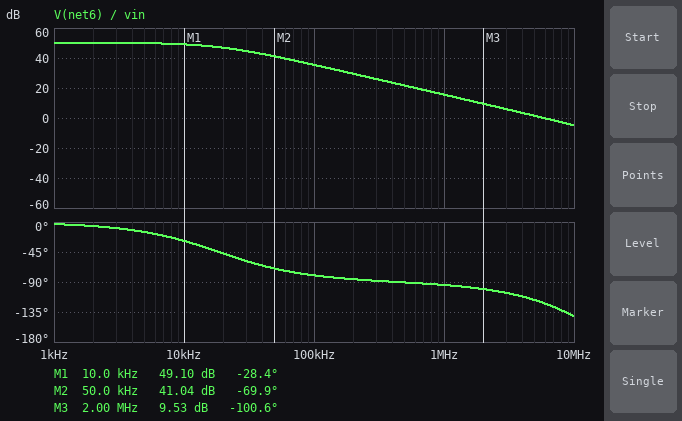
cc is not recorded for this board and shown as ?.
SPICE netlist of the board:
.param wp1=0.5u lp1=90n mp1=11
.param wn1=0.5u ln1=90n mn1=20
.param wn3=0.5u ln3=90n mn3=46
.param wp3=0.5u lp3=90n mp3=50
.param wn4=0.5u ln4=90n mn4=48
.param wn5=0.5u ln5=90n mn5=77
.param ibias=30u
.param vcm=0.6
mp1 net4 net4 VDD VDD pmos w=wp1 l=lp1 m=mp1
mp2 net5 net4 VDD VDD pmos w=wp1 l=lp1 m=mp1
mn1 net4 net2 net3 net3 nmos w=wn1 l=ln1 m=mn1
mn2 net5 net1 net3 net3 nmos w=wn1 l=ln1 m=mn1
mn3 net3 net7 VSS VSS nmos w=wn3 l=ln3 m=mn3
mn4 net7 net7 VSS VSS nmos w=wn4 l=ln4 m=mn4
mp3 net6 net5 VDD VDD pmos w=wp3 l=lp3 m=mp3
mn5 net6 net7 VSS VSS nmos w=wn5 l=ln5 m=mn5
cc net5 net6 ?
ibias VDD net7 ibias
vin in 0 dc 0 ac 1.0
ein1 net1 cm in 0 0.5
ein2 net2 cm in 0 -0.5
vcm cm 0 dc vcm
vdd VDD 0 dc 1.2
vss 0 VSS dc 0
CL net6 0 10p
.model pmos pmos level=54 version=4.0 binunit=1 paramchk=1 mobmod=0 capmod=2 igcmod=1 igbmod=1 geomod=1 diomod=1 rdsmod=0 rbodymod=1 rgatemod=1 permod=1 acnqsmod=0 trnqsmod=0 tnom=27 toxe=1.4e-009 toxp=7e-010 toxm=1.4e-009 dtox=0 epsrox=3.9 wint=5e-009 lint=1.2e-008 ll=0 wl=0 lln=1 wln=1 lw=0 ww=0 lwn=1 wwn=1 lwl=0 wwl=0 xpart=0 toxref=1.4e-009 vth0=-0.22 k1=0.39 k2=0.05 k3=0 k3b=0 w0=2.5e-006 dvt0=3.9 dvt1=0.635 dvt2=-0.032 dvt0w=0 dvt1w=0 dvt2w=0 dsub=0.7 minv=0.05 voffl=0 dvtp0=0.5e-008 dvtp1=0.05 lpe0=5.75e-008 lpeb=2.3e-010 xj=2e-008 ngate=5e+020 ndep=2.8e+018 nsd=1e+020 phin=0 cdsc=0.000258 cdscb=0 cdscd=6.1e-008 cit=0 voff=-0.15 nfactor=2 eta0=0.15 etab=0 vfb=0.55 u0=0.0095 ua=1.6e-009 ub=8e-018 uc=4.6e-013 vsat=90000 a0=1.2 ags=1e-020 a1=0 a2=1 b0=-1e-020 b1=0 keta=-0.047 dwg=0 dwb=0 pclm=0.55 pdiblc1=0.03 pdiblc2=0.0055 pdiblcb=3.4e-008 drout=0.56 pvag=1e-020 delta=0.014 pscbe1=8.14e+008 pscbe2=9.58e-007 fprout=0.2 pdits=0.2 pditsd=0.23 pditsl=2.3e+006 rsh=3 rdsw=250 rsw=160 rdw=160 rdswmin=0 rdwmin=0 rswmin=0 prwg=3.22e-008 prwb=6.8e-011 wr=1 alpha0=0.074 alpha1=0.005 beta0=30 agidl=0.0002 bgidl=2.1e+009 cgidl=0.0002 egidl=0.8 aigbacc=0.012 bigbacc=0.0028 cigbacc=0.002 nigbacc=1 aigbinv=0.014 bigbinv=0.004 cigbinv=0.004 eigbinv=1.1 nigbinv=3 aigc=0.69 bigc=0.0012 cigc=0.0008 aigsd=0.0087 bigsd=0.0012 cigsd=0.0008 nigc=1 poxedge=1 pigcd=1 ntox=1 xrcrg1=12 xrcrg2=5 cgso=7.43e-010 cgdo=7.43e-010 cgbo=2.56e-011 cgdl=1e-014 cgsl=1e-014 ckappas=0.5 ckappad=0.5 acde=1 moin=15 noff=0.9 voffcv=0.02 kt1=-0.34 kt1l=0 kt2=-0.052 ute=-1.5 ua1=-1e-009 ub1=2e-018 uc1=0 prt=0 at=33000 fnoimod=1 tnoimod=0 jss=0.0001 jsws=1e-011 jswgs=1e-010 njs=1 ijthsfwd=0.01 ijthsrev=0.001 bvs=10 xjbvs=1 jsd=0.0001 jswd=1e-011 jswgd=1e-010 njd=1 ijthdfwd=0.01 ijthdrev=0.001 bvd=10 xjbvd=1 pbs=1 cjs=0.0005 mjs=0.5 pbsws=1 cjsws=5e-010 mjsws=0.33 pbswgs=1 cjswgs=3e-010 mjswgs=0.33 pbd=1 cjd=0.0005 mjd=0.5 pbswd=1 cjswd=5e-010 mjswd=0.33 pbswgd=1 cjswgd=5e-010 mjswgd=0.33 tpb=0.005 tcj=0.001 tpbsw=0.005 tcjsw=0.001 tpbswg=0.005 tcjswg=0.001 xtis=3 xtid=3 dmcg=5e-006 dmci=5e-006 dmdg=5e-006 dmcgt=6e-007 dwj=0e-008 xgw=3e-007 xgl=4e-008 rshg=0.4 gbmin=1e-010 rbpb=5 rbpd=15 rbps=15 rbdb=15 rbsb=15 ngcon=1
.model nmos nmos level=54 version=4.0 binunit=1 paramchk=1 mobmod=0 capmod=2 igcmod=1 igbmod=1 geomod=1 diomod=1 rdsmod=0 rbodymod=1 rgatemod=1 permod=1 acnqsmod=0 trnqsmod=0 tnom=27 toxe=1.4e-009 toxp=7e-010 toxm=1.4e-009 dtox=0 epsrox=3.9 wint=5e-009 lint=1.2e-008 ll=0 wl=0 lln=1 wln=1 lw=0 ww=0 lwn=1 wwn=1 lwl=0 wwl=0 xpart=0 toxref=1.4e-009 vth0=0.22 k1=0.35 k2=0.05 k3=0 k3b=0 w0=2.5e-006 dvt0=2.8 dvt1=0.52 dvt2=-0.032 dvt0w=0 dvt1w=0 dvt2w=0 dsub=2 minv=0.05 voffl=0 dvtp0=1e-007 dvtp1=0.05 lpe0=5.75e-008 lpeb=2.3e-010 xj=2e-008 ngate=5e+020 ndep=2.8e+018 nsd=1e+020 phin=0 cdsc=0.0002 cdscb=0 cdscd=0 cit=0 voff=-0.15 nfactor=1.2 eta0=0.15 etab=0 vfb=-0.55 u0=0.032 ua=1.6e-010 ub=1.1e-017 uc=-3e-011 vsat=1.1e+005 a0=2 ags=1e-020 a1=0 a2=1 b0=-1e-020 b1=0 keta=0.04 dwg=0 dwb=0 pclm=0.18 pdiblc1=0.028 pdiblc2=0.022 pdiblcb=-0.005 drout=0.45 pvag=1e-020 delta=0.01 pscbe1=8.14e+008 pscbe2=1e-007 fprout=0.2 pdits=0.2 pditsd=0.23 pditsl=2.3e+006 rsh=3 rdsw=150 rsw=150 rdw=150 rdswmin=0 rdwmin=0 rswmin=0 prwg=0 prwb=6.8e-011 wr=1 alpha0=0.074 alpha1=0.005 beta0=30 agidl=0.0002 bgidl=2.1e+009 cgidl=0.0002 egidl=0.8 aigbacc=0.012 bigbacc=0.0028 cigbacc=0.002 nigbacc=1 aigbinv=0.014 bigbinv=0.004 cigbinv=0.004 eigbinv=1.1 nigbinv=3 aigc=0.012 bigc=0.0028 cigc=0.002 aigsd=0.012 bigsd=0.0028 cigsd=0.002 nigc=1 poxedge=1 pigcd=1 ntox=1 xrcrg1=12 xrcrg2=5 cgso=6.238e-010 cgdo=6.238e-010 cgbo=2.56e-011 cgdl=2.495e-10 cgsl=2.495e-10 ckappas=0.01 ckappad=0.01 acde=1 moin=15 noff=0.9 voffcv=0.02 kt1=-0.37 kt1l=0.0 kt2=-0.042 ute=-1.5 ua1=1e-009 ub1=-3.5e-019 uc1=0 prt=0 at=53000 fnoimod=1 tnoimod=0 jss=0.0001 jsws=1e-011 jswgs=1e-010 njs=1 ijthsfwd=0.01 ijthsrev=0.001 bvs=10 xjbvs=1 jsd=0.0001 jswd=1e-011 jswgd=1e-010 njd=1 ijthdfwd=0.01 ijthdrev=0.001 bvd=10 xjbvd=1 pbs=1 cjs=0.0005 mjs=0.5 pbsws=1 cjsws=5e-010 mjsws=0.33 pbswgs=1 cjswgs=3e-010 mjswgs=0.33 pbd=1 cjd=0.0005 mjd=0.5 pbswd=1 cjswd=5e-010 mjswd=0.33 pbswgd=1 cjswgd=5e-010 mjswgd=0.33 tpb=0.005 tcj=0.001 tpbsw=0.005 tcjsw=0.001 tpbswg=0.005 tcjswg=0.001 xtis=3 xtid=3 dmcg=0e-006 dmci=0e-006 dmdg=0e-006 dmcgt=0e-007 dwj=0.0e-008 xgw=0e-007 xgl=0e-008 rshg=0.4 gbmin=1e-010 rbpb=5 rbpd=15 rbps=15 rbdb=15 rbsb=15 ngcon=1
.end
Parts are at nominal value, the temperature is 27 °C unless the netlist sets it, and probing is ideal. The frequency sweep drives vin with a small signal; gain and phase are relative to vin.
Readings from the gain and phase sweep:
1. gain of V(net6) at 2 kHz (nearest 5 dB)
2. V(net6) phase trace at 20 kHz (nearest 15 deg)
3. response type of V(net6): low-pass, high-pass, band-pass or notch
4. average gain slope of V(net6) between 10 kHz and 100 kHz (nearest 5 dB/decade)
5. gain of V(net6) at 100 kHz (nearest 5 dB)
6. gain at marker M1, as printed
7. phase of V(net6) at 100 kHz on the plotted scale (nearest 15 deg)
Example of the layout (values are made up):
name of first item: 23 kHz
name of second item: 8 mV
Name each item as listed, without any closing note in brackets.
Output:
gain of V(net6) at 2 kHz: 50 dB
V(net6) phase trace at 20 kHz: -45 deg
response type of V(net6): low-pass, high-pass, band-pass or notch: low-pass
average gain slope of V(net6) between 10 kHz and 100 kHz: -15 dB/decade
gain of V(net6) at 100 kHz: 35 dB
gain at marker M1, as printed: 49.10 dB
phase of V(net6) at 100 kHz on the plotted scale: -75 deg
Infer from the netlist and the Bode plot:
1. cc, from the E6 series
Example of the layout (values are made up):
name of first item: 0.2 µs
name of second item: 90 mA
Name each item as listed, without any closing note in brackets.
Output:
cc, from the E6 series: 6.8 pF
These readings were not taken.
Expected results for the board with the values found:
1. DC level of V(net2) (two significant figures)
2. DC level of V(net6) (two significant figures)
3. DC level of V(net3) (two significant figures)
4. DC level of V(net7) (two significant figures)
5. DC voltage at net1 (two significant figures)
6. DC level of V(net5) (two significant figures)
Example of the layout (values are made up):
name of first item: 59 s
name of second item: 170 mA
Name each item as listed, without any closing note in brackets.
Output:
DC level of V(net2): 600 mV
DC level of V(net6): 760 mV
DC level of V(net3): 300 mV
DC level of V(net7): 300 mV
DC voltage at net1: 600 mV
DC level of V(net5): 830 mV
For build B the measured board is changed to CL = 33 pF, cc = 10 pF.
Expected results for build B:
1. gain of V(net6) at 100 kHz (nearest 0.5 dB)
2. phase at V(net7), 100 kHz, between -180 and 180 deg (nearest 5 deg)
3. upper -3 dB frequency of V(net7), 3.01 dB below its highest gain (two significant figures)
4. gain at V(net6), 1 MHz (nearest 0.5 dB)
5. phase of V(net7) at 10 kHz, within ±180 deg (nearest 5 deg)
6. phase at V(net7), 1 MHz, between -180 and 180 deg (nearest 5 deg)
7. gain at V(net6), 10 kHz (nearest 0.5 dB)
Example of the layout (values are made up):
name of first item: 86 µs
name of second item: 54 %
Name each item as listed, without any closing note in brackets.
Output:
gain of V(net6) at 100 kHz: 32.0 dB
phase at V(net7), 100 kHz, between -180 and 180 deg: -85 deg
upper -3 dB frequency of V(net7), 3.01 dB below its highest gain: 12 kHz
gain at V(net6), 1 MHz: 12.0 dB
phase of V(net7) at 10 kHz, within ±180 deg: -40 deg
phase at V(net7), 1 MHz, between -180 and 180 deg: -100 deg
gain at V(net6), 10 kHz: 48.0 dB
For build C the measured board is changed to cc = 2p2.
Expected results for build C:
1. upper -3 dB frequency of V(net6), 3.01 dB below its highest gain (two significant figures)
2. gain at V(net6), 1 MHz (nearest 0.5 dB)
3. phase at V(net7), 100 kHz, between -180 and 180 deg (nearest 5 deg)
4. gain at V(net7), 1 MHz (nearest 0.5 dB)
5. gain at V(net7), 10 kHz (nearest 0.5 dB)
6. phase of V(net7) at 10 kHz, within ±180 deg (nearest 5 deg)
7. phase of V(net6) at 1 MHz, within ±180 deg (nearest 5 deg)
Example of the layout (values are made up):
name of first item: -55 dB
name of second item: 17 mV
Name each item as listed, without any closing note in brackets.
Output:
upper -3 dB frequency of V(net6), 3.01 dB below its highest gain: 55 kHz
gain at V(net6), 1 MHz: 25.0 dB
phase at V(net7), 100 kHz, between -180 and 180 deg: -60 deg
gain at V(net7), 1 MHz: -22.0 dB
gain at V(net7), 10 kHz: 3.0 dB
phase of V(net7) at 10 kHz, within ±180 deg: -10 deg
phase of V(net6) at 1 MHz, within ±180 deg: -90 deg
